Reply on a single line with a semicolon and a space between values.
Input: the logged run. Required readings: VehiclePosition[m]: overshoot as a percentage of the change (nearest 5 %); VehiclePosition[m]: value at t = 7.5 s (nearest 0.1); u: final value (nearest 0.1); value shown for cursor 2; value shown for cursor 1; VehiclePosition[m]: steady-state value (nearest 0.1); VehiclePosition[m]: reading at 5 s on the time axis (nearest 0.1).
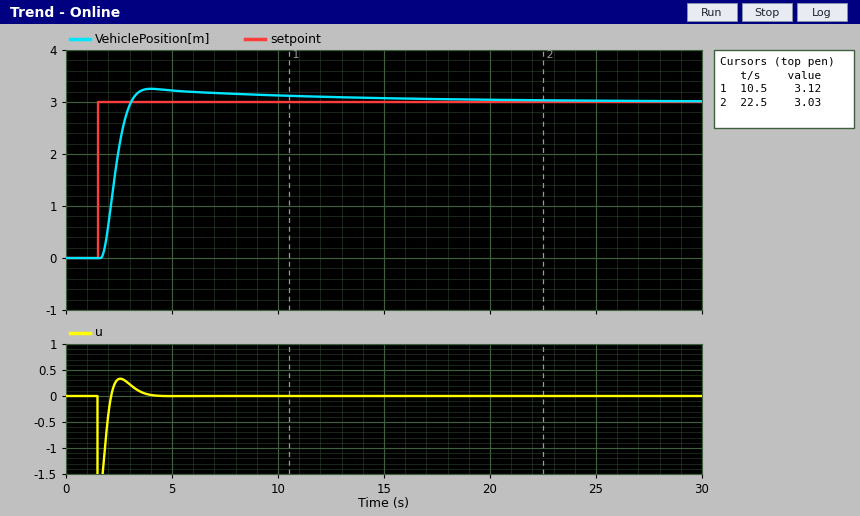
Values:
10 %; 3.2; 0.0; 3.03; 3.12; 3.0; 3.2
